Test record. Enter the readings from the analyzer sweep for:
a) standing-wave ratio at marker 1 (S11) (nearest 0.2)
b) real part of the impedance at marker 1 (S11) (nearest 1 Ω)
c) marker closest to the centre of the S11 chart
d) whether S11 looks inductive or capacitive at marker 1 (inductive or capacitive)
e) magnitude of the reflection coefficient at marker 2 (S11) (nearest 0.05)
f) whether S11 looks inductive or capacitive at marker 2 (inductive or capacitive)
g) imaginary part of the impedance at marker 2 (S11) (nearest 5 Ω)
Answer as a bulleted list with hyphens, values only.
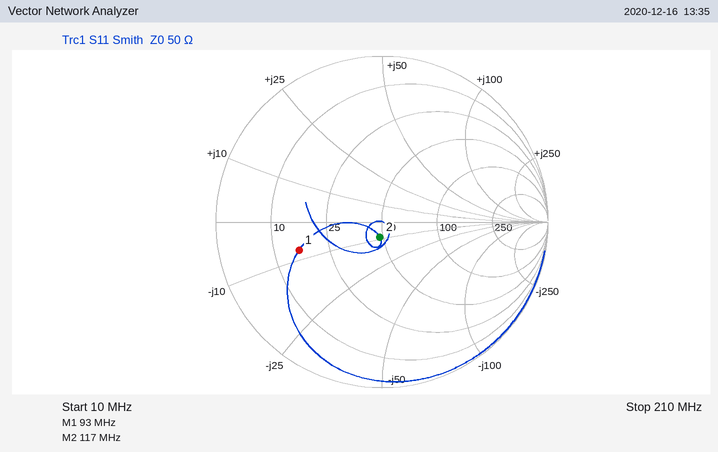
- 3.2
- 16 Ω
- marker 2
- capacitive
- 0.10
- capacitive
- -10 Ω
